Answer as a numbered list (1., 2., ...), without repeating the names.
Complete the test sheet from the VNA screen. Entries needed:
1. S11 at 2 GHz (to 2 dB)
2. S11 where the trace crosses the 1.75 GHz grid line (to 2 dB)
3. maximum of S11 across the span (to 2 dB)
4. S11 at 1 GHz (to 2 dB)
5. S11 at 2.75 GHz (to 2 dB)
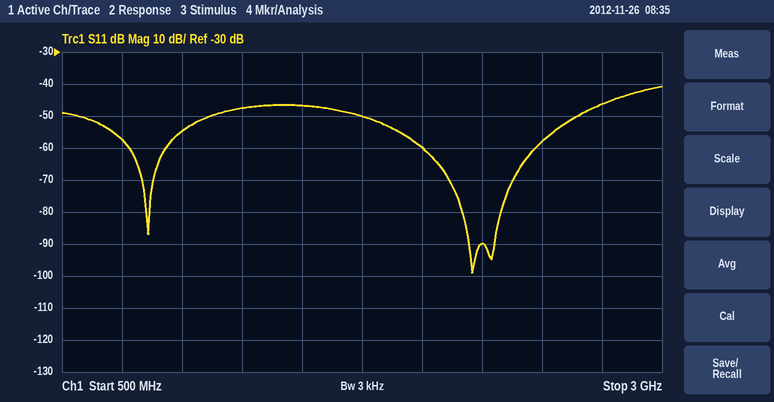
1. -60 dB
2. -50 dB
3. -40 dB
4. -54 dB
5. -46 dB
